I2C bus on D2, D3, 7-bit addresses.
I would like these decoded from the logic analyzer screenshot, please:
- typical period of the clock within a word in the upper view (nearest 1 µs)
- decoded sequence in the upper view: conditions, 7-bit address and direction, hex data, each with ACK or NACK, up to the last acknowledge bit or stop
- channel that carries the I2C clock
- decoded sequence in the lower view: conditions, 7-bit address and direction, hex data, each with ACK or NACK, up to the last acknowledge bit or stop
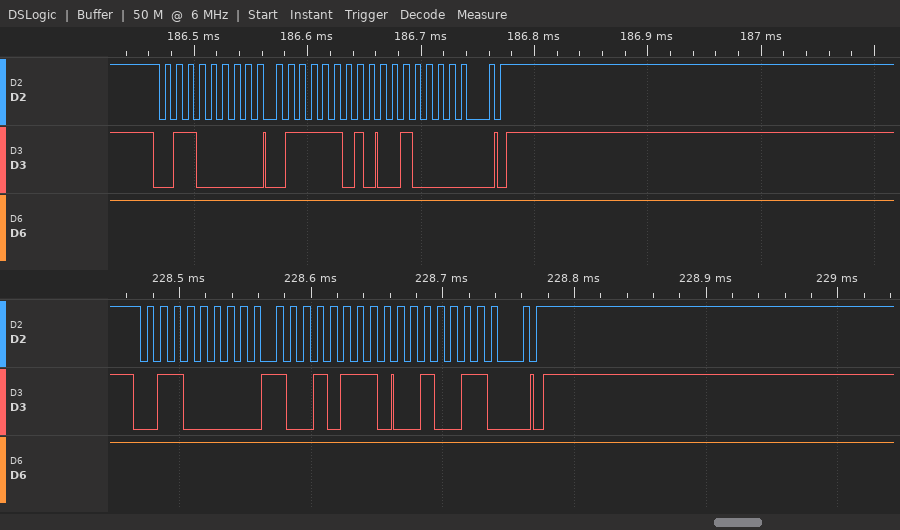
10 µs
start, address 30 write ACK, 7D ACK, 20 ACK, stop
D2
start, address 30 write ACK, 97 ACK, 26 ACK, stop
